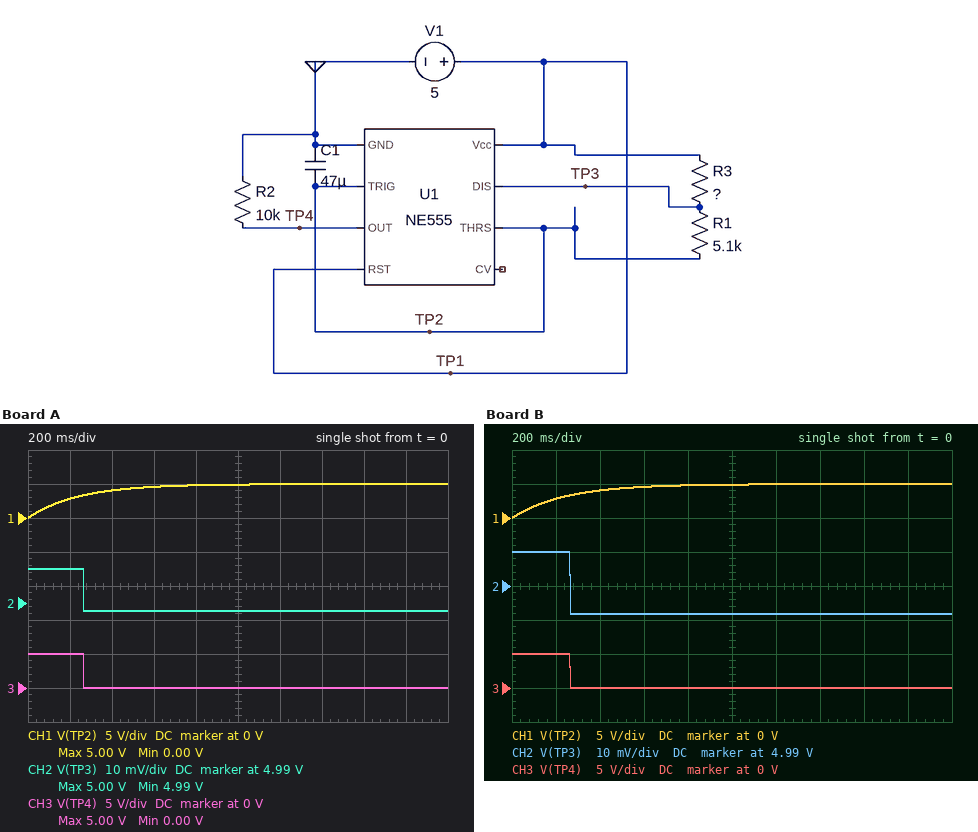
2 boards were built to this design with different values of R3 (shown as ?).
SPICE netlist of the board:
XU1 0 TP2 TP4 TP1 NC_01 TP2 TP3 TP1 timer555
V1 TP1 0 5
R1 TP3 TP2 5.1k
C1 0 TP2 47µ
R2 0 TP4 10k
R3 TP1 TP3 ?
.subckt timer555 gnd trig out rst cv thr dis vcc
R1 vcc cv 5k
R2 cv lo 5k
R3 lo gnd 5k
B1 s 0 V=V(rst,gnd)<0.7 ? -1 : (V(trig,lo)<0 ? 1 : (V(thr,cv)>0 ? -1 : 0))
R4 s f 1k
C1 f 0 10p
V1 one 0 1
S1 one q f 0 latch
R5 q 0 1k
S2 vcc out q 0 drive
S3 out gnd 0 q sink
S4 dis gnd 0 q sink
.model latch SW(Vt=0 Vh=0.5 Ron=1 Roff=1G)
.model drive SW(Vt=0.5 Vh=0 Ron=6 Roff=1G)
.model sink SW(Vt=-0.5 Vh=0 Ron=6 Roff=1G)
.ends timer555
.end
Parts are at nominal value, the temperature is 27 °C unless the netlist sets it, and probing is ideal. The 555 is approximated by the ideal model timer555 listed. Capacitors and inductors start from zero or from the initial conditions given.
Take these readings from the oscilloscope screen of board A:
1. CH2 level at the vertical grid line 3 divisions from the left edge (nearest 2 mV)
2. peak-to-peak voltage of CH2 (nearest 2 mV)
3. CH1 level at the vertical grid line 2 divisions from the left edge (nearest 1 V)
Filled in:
4.988 V
12 mV
4 V
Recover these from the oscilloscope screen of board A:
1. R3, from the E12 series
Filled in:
0.015 Ω
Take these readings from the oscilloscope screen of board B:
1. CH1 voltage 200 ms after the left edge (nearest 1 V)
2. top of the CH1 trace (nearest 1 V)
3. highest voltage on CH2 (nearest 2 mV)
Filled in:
3 V
5 V
5.000 V
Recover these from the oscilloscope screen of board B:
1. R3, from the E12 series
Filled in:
0.022 Ω
